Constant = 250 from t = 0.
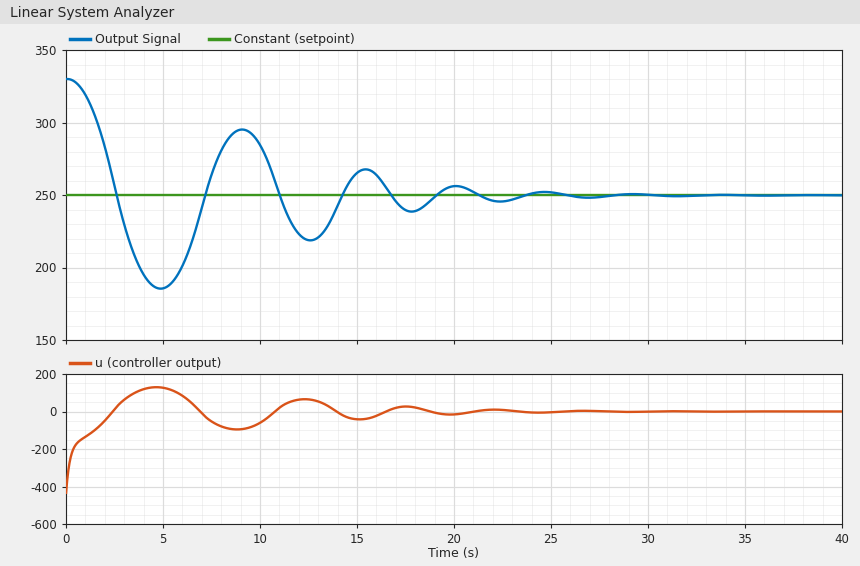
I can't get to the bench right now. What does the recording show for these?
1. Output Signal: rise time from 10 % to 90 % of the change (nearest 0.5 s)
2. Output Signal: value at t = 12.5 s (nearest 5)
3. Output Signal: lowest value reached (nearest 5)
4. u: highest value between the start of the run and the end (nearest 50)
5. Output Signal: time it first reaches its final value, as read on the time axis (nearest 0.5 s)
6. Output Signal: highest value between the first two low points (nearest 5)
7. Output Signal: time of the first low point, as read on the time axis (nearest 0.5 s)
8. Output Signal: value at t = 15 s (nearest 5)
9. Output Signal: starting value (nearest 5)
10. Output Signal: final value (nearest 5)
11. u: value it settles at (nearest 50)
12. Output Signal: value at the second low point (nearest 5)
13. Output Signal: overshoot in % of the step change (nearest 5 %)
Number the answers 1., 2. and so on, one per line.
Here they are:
1. 1.5 s
2. 220
3. 185
4. 150
5. 2.5 s
6. 295
7. 5.0 s
8. 265
9. 330
10. 250
11. 0
12. 220
13. 80 %
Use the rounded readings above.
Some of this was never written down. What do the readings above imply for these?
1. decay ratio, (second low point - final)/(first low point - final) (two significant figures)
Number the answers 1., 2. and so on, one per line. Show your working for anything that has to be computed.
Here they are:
1. (220 - 250) / (185 - 250) = 0.46
